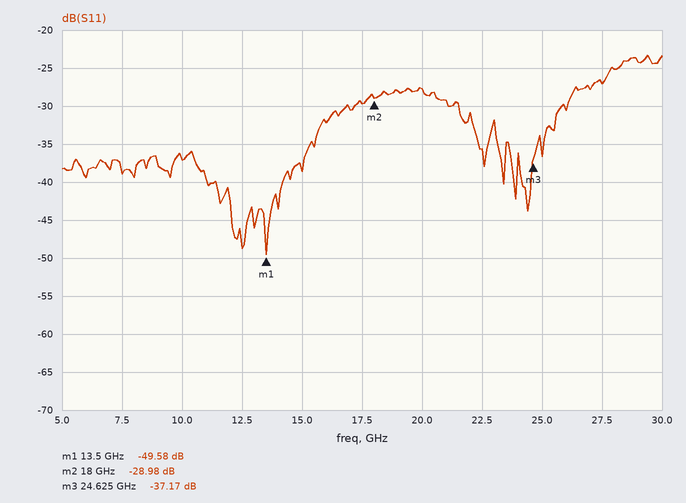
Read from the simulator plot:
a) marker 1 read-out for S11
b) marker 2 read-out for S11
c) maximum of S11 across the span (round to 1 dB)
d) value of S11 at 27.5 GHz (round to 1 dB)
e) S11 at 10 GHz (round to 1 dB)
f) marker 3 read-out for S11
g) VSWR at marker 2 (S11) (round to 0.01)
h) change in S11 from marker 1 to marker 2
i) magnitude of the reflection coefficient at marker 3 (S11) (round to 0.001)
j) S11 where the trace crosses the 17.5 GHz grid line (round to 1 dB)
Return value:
-49.58 dB
-28.98 dB
-23 dB
-27 dB
-37 dB
-37.17 dB
1.07
20.60 dB
0.014
-30 dB
